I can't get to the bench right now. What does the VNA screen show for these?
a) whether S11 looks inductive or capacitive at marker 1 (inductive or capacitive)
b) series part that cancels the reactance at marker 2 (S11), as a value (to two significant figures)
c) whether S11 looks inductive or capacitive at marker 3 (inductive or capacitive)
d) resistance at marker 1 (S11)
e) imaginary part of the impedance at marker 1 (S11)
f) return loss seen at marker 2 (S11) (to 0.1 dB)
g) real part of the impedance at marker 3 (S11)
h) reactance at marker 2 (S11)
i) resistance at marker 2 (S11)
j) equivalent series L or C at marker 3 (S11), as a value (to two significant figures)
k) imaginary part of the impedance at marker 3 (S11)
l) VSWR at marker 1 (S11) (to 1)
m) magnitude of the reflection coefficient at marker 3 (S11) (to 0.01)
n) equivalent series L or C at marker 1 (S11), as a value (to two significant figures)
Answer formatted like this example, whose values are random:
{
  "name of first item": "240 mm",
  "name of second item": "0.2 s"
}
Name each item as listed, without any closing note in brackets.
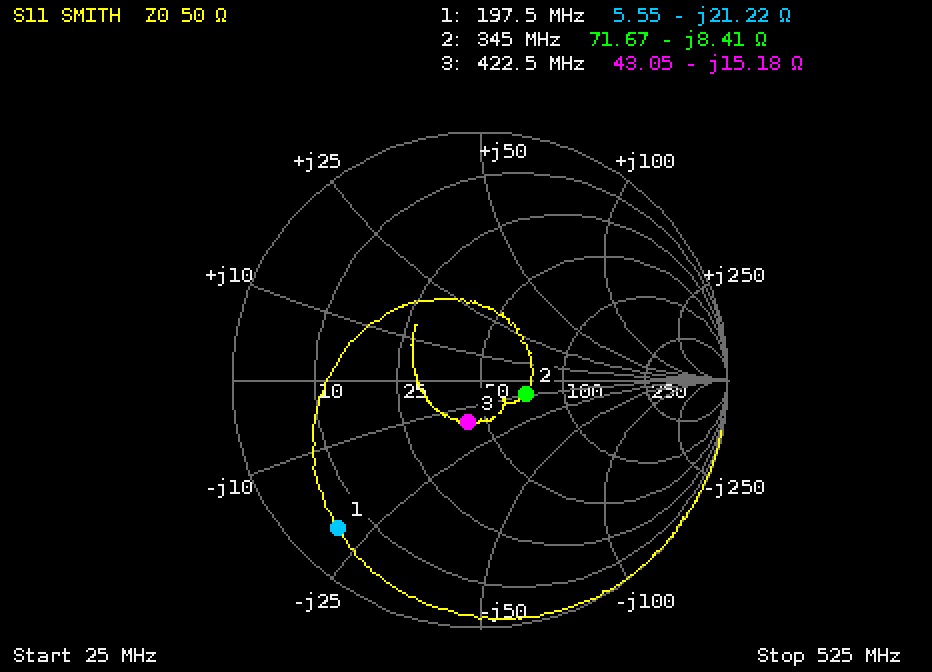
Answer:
{
  "whether S11 looks inductive or capacitive at marker 1": "capacitive",
  "series part that cancels the reactance at marker 2 (S11), as a value": "3.9 nH",
  "whether S11 looks inductive or capacitive at marker 3": "capacitive",
  "resistance at marker 1": "5.55 Ω",
  "imaginary part of the impedance at marker 1": "-21.22 Ω",
  "return loss seen at marker 2 (S11)": "14.4 dB",
  "real part of the impedance at marker 3": "43.05 Ω",
  "reactance at marker 2": "-8.41 Ω",
  "resistance at marker 2": "71.67 Ω",
  "equivalent series L or C at marker 3 (S11), as a value": "25 pF",
  "imaginary part of the impedance at marker 3": "-15.18 Ω",
  "VSWR at marker 1 (S11)": "11",
  "magnitude of the reflection coefficient at marker 3 (S11)": "0.18",
  "equivalent series L or C at marker 1 (S11), as a value": "38 pF"
}
